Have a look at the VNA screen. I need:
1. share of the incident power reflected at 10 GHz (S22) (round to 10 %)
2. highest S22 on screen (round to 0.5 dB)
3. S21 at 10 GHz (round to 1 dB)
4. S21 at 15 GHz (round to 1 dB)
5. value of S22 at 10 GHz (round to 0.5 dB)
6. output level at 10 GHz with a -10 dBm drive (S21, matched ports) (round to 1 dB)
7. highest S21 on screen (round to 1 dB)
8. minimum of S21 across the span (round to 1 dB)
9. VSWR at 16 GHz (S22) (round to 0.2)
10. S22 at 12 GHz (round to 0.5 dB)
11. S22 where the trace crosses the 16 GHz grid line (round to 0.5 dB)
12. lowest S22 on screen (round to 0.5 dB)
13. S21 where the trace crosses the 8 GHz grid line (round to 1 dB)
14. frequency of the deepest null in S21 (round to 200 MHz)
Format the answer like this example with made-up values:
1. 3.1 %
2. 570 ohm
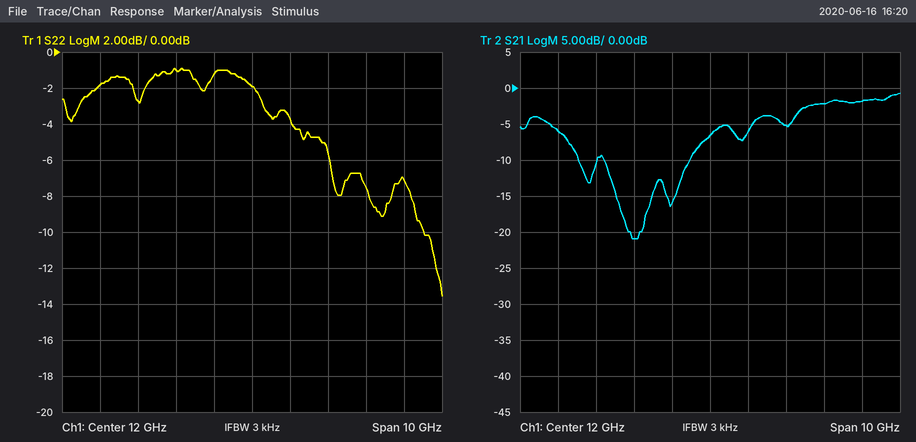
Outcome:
1. 80 %
2. -1.0 dB
3. -21 dB
4. -2 dB
5. -1.0 dB
6. -31 dBm
7. -1 dB
8. -21 dB
9. 2.6
10. -2.0 dB
11. -7.0 dB
12. -13.5 dB
13. -6 dB
14. 10.0 GHz
